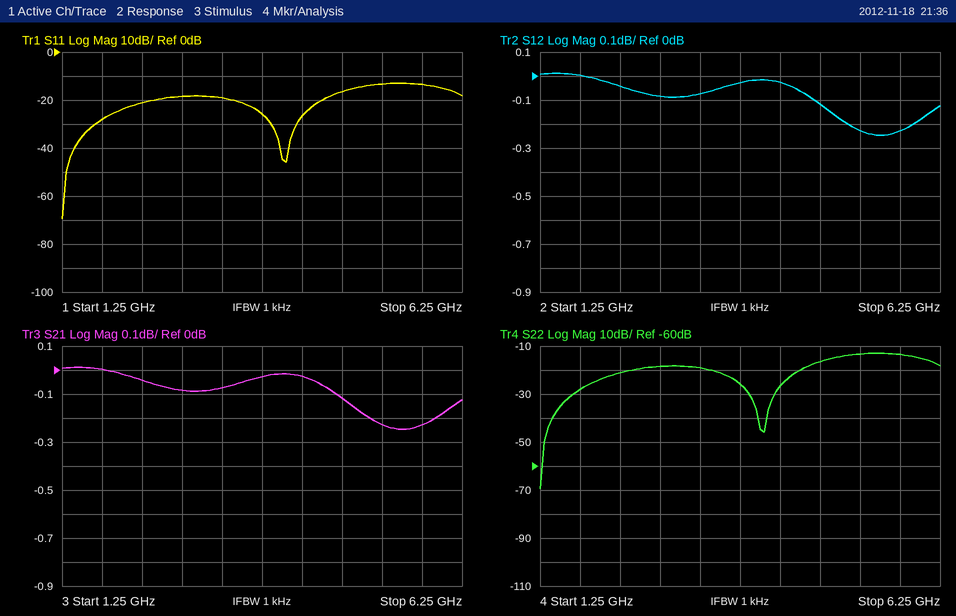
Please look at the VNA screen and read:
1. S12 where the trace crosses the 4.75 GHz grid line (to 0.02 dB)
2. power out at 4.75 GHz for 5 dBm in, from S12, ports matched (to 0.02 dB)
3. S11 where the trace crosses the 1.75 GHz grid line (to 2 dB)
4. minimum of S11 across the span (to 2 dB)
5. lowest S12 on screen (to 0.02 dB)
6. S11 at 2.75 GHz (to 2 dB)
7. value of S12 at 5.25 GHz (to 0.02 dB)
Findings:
-0.12 dB
4.88 dBm
-28 dB
-70 dB
-0.24 dB
-18 dB
-0.22 dB
